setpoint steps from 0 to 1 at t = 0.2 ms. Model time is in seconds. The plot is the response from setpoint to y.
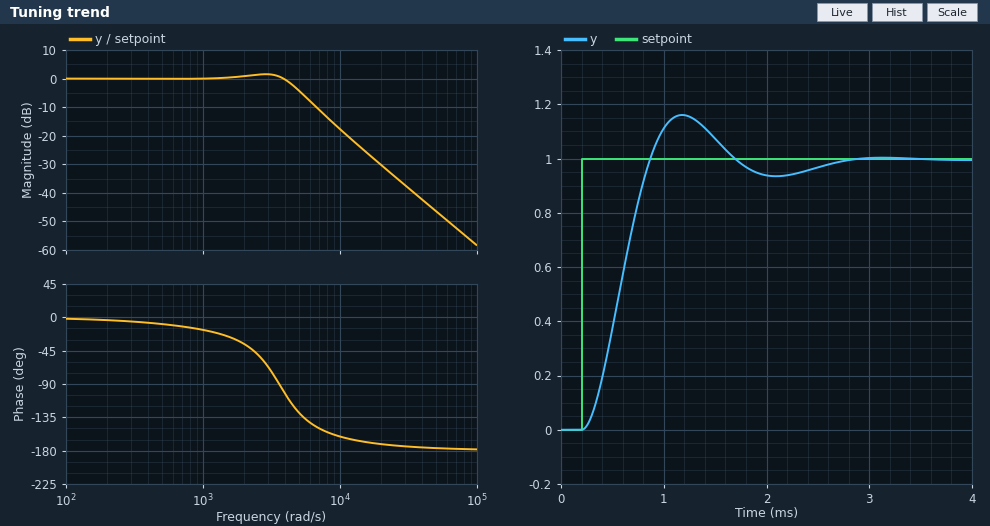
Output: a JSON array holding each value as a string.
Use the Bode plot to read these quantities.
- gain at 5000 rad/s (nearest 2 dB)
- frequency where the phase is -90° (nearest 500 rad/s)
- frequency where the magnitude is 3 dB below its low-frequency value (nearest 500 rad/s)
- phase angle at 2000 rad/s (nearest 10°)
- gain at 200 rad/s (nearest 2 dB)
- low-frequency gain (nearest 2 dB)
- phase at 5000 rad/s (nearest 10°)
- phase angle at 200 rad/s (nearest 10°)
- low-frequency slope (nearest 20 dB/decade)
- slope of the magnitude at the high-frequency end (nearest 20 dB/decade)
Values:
["-4 dB", "3500 rad/s", "4500 rad/s", "-40°", "0 dB", "0 dB", "-130°", "0°", "0 dB/decade", "-40 dB/decade"]
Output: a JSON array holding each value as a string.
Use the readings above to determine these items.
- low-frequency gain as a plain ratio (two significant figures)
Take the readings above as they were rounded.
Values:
["1.0"]
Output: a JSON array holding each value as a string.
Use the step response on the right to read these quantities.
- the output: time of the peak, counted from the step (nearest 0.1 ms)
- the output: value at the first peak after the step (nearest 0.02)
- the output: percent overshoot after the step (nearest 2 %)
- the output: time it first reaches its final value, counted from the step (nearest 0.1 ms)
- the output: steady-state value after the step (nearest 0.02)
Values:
["1.0 ms", "1.16", "16 %", "0.7 ms", "1.00"]
